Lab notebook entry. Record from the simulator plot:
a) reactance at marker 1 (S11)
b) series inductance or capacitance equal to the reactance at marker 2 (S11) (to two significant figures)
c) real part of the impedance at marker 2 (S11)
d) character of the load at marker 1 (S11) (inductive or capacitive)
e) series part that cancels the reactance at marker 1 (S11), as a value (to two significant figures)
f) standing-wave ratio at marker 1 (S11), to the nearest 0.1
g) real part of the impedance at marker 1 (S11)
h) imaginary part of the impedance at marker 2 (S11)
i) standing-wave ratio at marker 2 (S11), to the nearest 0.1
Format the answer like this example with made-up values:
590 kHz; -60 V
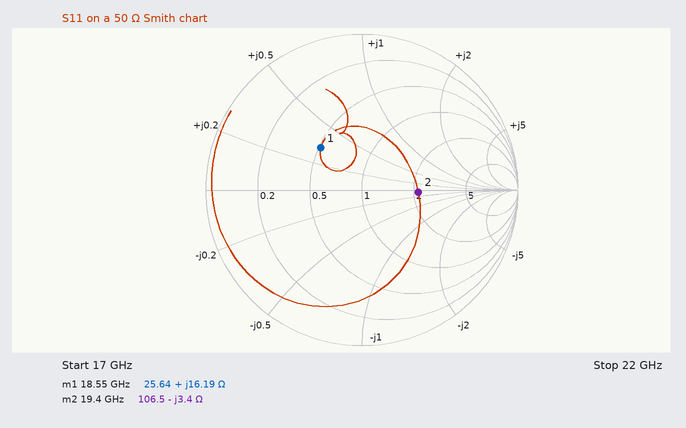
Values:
+16.19 Ω; 2.4 pF; 106.5 Ω; inductive; 530 fF; 2.2; 25.64 Ω; -3.4 Ω; 2.1
